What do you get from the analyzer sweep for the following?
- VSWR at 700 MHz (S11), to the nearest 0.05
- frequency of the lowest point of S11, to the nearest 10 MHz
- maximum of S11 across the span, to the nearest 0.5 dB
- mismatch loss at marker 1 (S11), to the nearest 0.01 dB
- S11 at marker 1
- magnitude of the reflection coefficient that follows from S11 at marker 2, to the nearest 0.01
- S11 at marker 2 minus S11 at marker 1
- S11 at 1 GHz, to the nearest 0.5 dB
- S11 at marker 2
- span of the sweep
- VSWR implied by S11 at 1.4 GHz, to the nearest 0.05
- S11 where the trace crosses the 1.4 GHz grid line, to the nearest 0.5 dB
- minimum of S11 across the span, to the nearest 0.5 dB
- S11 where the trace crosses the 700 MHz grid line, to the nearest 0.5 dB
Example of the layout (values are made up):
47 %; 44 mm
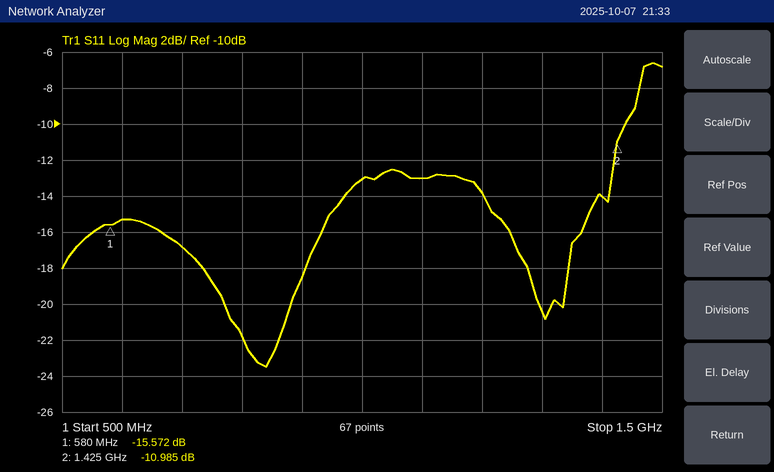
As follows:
1.35; 840 MHz; -6.5 dB; 0.12 dB; -15.572 dB; 0.28; 4.587 dB; -13.0 dB; -10.985 dB; 1 GHz; 1.50; -14.0 dB; -23.5 dB; -17.0 dB
